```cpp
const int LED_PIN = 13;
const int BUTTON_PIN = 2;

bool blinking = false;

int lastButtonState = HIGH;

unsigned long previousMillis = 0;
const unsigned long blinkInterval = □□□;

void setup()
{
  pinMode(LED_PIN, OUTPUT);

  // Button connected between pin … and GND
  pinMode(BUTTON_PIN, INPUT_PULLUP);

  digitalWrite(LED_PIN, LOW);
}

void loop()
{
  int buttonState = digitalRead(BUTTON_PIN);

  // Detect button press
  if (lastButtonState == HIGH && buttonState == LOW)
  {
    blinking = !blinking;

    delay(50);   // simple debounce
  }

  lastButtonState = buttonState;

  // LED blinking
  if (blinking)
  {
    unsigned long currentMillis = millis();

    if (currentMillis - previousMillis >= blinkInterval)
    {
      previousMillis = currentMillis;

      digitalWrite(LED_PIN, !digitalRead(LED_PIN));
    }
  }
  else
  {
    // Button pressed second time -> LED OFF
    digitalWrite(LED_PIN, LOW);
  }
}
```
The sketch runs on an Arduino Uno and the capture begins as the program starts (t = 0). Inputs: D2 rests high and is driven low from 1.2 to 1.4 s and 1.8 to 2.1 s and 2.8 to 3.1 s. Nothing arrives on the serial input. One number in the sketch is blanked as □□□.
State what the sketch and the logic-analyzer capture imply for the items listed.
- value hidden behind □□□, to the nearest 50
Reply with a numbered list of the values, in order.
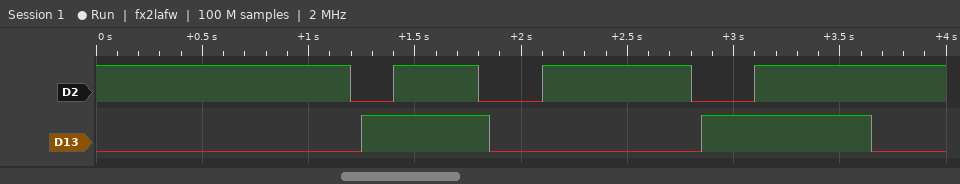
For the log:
1. 800
